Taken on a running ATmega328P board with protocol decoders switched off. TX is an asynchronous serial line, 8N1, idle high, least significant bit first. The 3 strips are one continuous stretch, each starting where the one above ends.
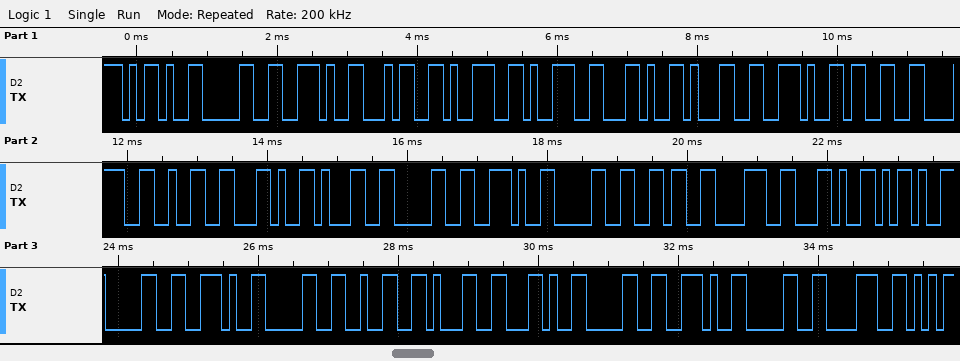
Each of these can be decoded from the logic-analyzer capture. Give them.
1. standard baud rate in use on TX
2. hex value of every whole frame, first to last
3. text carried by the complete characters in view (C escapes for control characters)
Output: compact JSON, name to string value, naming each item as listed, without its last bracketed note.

{"standard baud rate in use on TX": "9600 baud", "hex value of every whole frame, first to last": "2D 30 2E 34 39 39 2C 31 2E 33 38 32 2C 31 30 2E 30 36 38 2C 2D 30 2E 30 32 31 2C 30 2E 30 38", "text carried by the complete characters in view": "\"-0.499,1.382,10.068,-0.021,0.08\""}
